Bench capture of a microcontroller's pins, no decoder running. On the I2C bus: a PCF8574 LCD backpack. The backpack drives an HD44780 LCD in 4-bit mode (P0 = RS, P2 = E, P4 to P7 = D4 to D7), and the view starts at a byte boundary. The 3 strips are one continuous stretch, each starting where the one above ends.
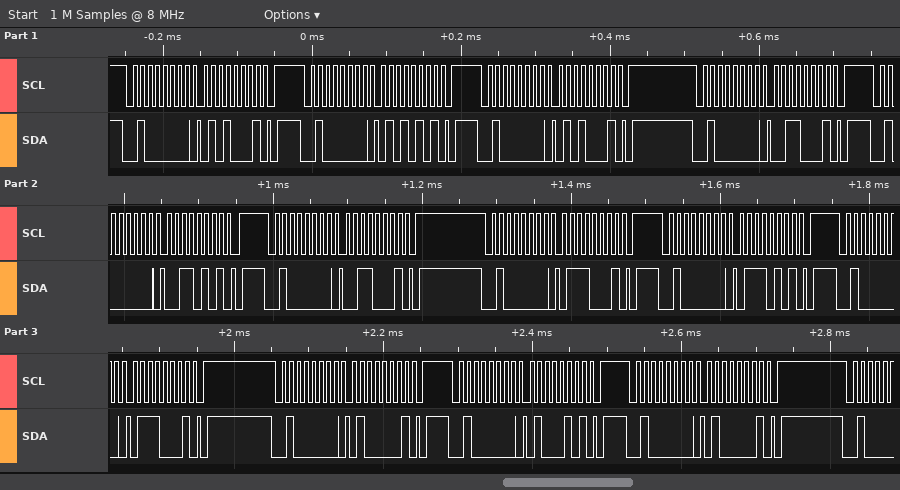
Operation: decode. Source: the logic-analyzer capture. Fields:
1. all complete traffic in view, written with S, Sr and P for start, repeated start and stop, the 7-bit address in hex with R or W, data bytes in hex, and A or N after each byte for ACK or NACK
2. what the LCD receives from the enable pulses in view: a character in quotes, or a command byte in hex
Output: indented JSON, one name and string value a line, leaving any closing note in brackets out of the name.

{
  "all complete traffic in view, written with S, Sr and P for start, repeated start and stop, the 7-bit address in hex with R or W, data bytes in hex, and A or N after each byte for ACK or NACK": "S 20W A 51 A P S 20W A 55 A P S 20W A 51 A P S 20W A 31 A P S 20W A 35 A P S 20W A 31 A P S 20W A 71 A P S 20W A 75 A P S 20W A 71 A P S 20W A 41 A P S 20W A 45 A P S 20W A 41 A P",
  "what the LCD receives from the enable pulses in view: a character in quotes, or a command byte in hex": "'S' 't'"
}
